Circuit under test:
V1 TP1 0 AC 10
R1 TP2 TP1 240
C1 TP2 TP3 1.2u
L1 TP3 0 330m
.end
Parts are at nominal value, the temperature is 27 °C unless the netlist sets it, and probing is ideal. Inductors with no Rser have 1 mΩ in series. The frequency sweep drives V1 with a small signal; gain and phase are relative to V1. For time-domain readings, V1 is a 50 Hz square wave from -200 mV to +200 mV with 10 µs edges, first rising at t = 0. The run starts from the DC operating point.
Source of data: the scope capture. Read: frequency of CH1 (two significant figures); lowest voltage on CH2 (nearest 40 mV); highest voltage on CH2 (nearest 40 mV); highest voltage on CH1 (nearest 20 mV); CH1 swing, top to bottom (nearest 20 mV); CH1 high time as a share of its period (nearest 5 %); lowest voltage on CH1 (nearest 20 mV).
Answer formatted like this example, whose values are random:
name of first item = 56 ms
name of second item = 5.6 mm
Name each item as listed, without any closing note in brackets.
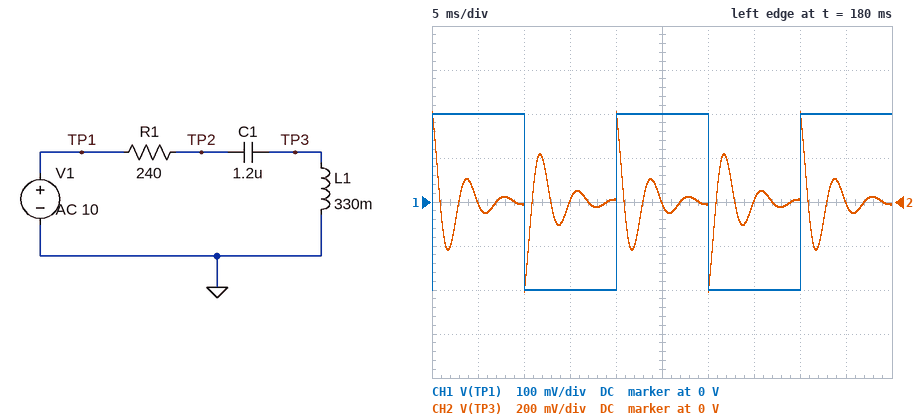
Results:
frequency of CH1 = 50 Hz
lowest voltage on CH2 = -400 mV
highest voltage on CH2 = 400 mV
highest voltage on CH1 = 200 mV
CH1 swing, top to bottom = 400 mV
CH1 high time as a share of its period = 50 %
lowest voltage on CH1 = -200 mV
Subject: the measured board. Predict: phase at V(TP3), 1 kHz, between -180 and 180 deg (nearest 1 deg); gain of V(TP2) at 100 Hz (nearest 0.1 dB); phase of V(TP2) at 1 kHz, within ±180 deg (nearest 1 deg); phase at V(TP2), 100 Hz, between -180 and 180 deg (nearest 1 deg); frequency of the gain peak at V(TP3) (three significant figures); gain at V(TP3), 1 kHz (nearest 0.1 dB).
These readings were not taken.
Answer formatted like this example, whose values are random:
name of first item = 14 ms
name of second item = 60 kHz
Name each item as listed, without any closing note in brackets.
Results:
phase at V(TP3), 1 kHz, between -180 and 180 deg = 7 deg
gain of V(TP2) at 100 Hz = -0.2 dB
phase of V(TP2) at 1 kHz, within ±180 deg = 7 deg
phase at V(TP2), 100 Hz, between -180 and 180 deg = -12 deg
frequency of the gain peak at V(TP3) = 267 Hz
gain at V(TP3), 1 kHz = 0.5 dB
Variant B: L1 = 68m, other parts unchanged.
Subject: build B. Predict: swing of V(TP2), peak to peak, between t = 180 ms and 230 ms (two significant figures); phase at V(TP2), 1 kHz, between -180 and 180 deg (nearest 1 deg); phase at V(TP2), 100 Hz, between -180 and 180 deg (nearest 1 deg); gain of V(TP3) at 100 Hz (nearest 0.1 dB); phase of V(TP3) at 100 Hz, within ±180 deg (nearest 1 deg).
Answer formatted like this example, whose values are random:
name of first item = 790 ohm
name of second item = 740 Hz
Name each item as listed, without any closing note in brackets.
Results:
swing of V(TP2), peak to peak, between t = 180 ms and 230 ms = 470 mV
phase at V(TP2), 1 kHz, between -180 and 180 deg = 39 deg
phase at V(TP2), 100 Hz, between -180 and 180 deg = -11 deg
gain of V(TP3) at 100 Hz = -29.7 dB
phase of V(TP3) at 100 Hz, within ±180 deg = 169 deg
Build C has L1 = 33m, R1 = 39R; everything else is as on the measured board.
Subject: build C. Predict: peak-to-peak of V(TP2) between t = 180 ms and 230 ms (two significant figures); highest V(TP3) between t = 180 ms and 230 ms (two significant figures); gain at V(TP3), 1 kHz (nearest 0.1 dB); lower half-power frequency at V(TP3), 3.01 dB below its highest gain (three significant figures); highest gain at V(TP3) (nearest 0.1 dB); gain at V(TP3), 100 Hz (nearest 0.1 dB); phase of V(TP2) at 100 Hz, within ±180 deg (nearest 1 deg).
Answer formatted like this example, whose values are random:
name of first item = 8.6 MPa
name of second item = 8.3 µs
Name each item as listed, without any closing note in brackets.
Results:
peak-to-peak of V(TP2) between t = 180 ms and 230 ms = 510 mV
highest V(TP3) between t = 180 ms and 230 ms = 400 mV
gain at V(TP3), 1 kHz = 7.8 dB
lower half-power frequency at V(TP3), 3.01 dB below its highest gain = 728 Hz
highest gain at V(TP3) = 12.6 dB
gain at V(TP3), 100 Hz = -36.0 dB
phase of V(TP2) at 100 Hz, within ±180 deg = -2 deg
